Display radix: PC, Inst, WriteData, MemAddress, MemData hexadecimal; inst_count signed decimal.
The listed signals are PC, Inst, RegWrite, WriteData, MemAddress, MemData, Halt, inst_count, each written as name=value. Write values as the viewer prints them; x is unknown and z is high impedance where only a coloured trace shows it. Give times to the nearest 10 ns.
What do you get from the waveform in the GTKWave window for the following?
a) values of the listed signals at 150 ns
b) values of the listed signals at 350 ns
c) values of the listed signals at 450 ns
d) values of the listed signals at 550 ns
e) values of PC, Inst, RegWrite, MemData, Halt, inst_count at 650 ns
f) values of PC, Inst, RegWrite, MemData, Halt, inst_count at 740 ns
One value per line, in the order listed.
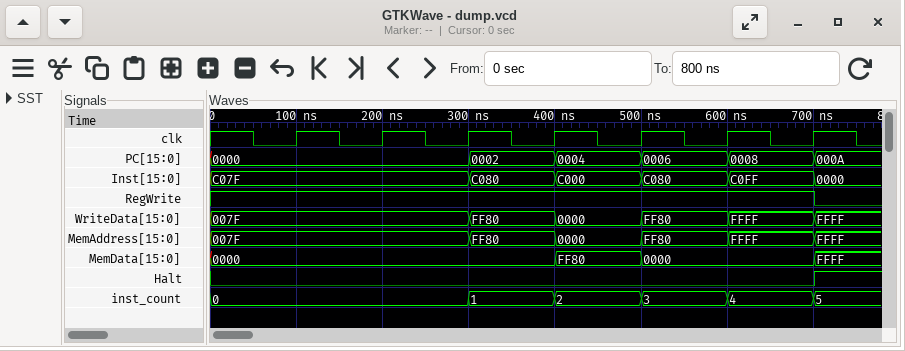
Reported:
PC=0000, Inst=C07F, RegWrite=1, WriteData=007F, MemAddress=007F, MemData=0000, Halt=0, inst_count=0
PC=0002, Inst=C080, RegWrite=1, WriteData=FF80, MemAddress=FF80, MemData=0000, Halt=0, inst_count=1
PC=0004, Inst=C000, RegWrite=1, WriteData=0000, MemAddress=0000, MemData=FF80, Halt=0, inst_count=2
PC=0006, Inst=C080, RegWrite=1, WriteData=FF80, MemAddress=FF80, MemData=0000, Halt=0, inst_count=3
PC=0008, Inst=C0FF, RegWrite=1, MemData=0000, Halt=0, inst_count=4
PC=000A, Inst=0000, RegWrite=0, MemData=FFFF, Halt=1, inst_count=5
